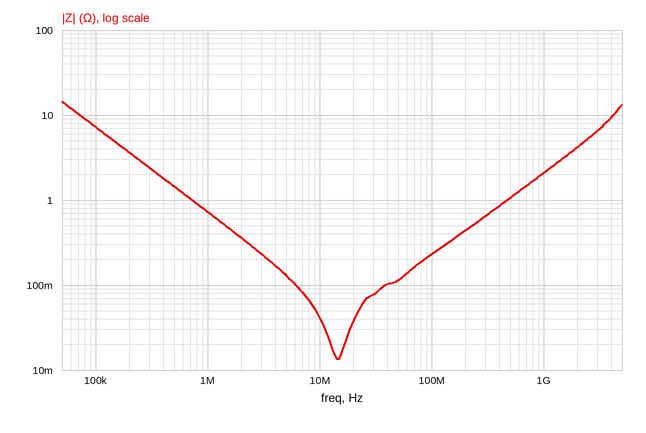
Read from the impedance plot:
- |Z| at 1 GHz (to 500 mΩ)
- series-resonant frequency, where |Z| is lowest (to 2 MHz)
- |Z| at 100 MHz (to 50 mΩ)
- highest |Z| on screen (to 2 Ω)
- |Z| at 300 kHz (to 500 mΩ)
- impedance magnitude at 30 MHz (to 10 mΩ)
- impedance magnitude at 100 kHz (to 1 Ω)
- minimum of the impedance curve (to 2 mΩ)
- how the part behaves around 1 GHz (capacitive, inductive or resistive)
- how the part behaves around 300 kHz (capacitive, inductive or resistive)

2.0 Ω
14 MHz
250 mΩ
14 Ω
2.5 Ω
80 mΩ
7 Ω
14 mΩ
inductive
capacitive
